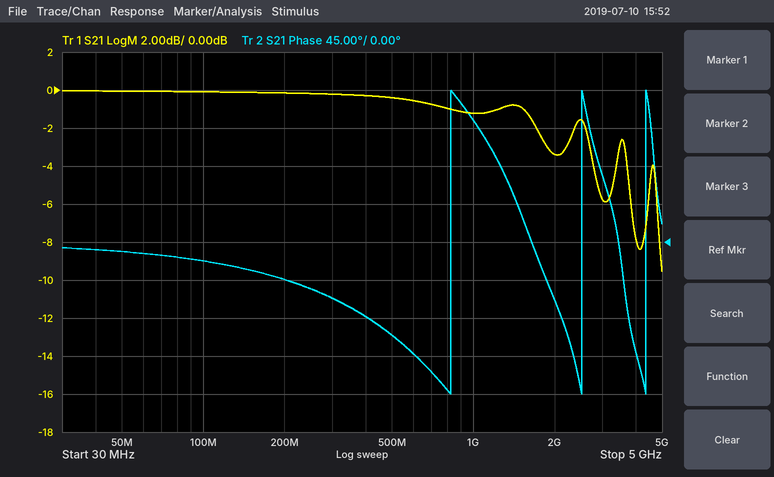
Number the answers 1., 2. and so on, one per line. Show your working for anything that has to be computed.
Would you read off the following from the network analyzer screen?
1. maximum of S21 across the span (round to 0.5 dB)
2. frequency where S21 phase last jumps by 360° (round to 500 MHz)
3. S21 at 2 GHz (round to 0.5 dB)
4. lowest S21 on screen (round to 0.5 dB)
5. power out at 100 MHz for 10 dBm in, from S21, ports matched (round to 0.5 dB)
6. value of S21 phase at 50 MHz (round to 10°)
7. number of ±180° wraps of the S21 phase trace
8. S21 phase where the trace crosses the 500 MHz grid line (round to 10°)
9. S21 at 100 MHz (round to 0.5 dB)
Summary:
1. 0.0 dB
2. 4.5 GHz
3. -3.5 dB
4. -9.5 dB
5. 10 dBm + (0.0 dB) = 10.0 dBm
6. -10°
7. 3
8. -110°
9. 0.0 dB
